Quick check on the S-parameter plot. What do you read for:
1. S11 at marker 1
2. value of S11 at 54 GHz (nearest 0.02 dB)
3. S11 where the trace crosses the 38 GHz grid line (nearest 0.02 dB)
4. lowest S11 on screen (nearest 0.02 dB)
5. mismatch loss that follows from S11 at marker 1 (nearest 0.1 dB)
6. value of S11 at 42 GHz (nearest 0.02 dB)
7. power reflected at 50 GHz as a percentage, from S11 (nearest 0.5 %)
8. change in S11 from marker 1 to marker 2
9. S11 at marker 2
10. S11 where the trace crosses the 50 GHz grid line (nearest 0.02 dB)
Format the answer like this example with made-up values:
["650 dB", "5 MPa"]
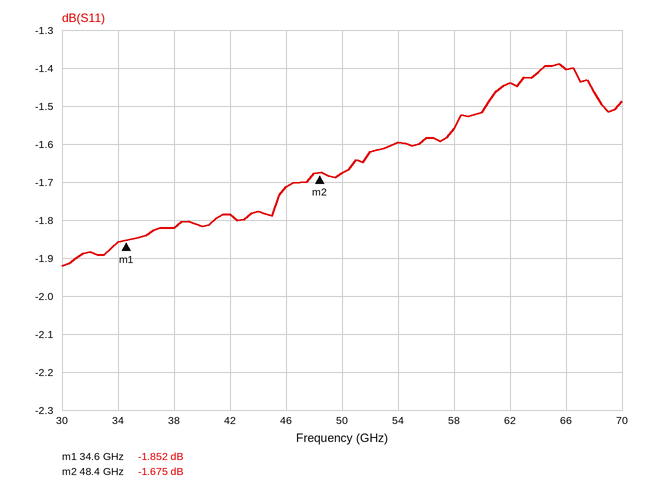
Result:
["-1.852 dB", "-1.60 dB", "-1.82 dB", "-1.92 dB", "4.6 dB", "-1.78 dB", "68.0 %", "0.177 dB", "-1.675 dB", "-1.68 dB"]
